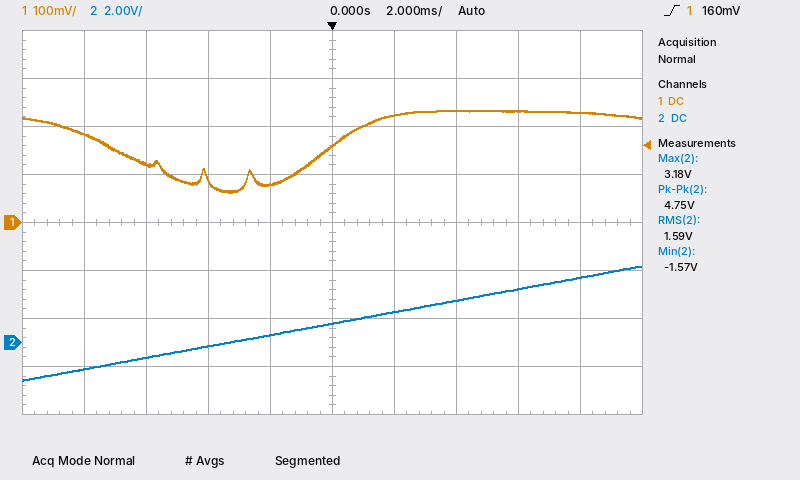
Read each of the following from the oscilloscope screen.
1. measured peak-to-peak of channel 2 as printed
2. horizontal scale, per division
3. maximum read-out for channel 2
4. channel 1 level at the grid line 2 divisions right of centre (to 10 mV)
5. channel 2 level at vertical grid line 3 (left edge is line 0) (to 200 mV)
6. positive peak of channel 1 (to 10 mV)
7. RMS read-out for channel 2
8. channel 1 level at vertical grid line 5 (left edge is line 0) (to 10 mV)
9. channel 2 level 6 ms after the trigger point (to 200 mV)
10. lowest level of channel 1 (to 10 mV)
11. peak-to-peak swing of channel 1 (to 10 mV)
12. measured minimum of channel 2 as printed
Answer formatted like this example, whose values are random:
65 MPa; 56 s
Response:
4.75 V; 2 ms; 3.18 V; 230 mV; -200 mV; 230 mV; 1.59 V; 160 mV; 2.2 V; 60 mV; 170 mV; -1.57 V
